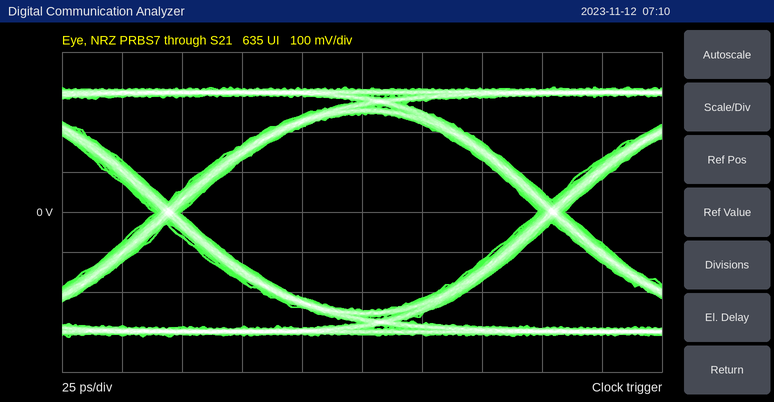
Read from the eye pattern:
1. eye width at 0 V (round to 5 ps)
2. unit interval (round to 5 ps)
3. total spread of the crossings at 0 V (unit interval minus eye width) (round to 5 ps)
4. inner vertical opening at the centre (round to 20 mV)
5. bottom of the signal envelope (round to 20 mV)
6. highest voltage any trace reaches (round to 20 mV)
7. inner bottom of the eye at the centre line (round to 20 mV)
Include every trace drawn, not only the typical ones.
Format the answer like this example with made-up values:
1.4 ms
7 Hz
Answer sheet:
150 ps
160 ps
10 ps
500 mV
-320 mV
320 mV
-240 mV
